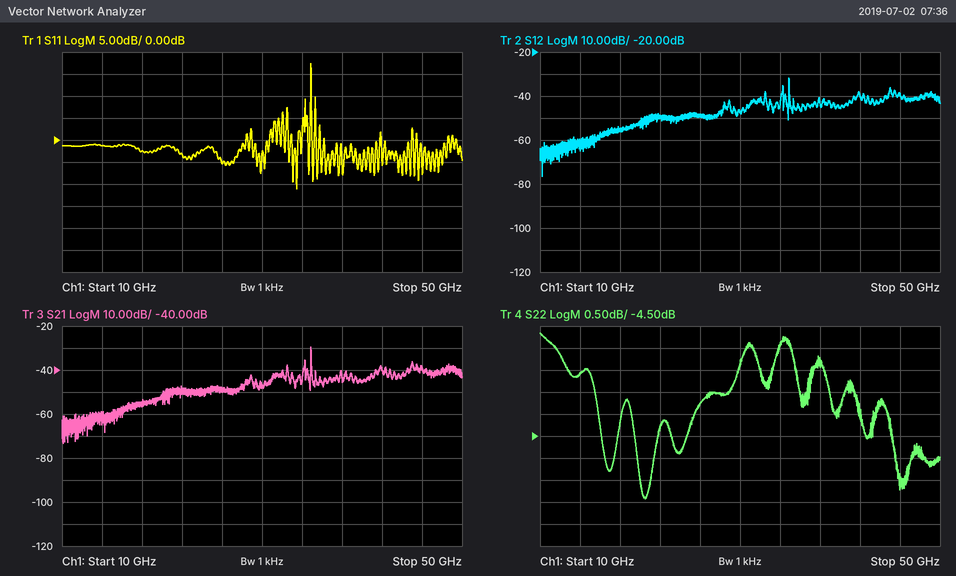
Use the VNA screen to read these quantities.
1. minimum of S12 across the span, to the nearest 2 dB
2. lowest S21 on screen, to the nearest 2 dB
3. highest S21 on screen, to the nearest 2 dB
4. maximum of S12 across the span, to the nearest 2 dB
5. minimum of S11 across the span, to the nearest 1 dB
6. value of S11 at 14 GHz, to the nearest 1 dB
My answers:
-76 dB
-74 dB
-30 dB
-32 dB
-11 dB
-1 dB
